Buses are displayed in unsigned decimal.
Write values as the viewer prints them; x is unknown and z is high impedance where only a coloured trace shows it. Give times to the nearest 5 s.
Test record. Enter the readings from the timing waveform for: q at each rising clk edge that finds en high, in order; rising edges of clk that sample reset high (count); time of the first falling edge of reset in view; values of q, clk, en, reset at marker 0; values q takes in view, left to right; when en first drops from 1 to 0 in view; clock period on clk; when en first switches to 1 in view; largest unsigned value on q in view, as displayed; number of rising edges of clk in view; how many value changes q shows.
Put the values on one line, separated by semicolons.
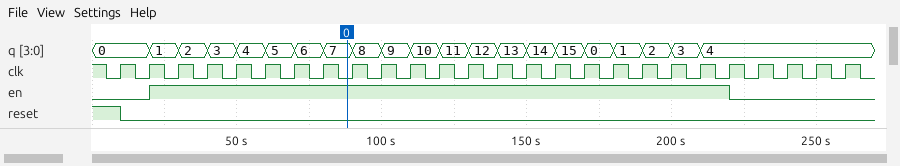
1, 2, 3, 4, 5, 6, 7, 8, 9, 10, 11, 12, 13, 14, 15, 0, 1, 2, 3, 4; 1; 10 s; q=7, clk=0, en=1, reset=0; 0, 1, 2, 3, 4, 5, 6, 7, 8, 9, 10, 11, 12, 13, 14, 15, 0, 1, 2, 3, 4; 220 s; 10 s; 20 s; 15; 26; 20
